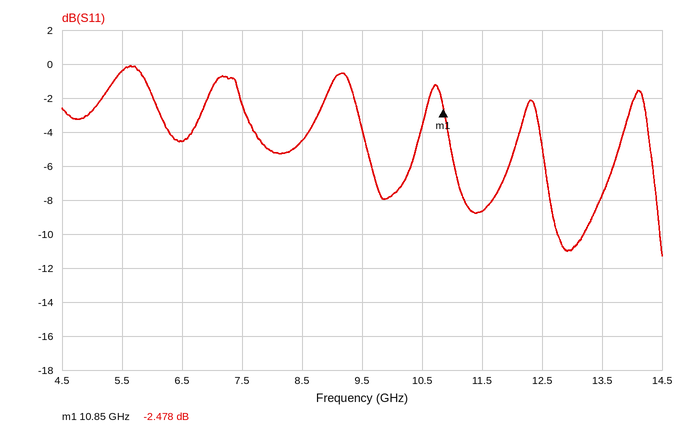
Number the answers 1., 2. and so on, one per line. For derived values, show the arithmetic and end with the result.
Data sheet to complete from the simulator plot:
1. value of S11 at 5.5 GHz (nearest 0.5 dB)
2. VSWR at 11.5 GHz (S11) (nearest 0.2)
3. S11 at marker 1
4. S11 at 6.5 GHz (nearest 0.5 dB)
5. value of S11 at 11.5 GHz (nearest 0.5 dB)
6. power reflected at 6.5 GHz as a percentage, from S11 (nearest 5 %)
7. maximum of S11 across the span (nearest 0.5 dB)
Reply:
1. -0.5 dB
2. |Γ| = 10^(-8.5/20) = 0.3758; VSWR = (1 + 0.3758)/(1 − 0.3758) ≈ 2.2
3. -2.478 dB
4. -4.5 dB
5. -8.5 dB
6. 10^(-4.5/10) ≈ 35 %
7. 0.0 dB
